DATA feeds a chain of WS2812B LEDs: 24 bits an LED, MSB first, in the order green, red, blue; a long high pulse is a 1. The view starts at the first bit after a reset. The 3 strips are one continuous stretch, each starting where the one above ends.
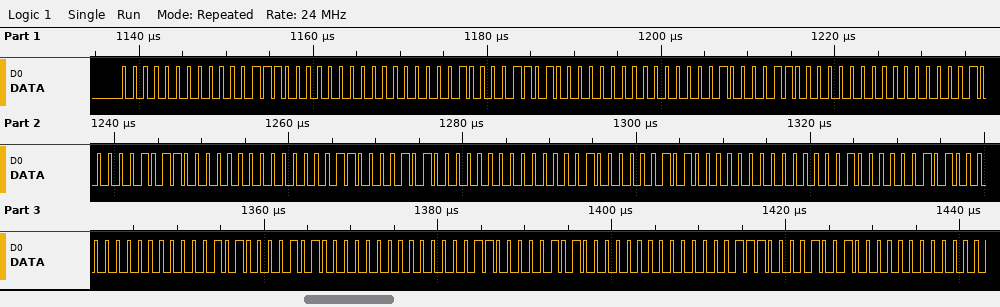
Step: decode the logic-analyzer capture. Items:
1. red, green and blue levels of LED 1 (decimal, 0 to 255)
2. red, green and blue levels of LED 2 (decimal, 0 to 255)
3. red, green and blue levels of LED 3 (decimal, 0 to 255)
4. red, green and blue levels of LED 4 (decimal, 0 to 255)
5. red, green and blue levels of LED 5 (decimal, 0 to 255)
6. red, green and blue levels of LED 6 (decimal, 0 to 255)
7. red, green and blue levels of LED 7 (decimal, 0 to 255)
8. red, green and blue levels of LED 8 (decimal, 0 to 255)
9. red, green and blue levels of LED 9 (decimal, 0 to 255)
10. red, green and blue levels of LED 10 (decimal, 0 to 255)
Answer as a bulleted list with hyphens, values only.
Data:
- 14, 0, 0
- 13, 1, 0
- 12, 1, 0
- 11, 2, 0
- 10, 3, 0
- 10, 4, 0
- 10, 4, 0
- 10, 5, 0
- 10, 6, 0
- 9, 7, 0
